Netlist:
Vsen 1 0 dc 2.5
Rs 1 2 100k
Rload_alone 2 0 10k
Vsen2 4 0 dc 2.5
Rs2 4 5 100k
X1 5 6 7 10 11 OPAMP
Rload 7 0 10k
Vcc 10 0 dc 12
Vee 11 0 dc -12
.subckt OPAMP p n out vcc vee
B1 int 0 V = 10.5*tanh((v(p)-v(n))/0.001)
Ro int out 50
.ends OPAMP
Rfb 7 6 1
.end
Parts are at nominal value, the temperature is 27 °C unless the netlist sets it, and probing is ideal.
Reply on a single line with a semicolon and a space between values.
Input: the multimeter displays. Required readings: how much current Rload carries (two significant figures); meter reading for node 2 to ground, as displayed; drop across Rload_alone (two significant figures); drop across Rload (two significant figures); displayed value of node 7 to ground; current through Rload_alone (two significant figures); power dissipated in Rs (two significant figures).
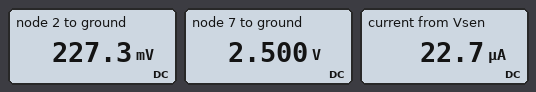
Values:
250 µA; 227.3 mV; 230 mV; 2.5 V; 2.500 V; 23 µA; 52 µW
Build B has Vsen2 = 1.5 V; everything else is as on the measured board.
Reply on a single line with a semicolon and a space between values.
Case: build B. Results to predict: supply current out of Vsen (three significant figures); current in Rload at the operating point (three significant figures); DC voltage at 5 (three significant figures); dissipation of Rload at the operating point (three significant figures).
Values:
22.7 µA; 150 µA; 1.50 V; 225 µW
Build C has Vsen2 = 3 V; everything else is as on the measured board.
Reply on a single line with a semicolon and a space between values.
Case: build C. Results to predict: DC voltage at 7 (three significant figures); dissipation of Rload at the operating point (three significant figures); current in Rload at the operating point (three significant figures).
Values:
3.00 V; 900 µW; 300 µA
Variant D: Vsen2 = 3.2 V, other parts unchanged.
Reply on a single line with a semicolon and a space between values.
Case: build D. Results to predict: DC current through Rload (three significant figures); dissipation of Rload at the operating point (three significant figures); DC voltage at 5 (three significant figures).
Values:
320 µA; 1.02 mW; 3.20 V
